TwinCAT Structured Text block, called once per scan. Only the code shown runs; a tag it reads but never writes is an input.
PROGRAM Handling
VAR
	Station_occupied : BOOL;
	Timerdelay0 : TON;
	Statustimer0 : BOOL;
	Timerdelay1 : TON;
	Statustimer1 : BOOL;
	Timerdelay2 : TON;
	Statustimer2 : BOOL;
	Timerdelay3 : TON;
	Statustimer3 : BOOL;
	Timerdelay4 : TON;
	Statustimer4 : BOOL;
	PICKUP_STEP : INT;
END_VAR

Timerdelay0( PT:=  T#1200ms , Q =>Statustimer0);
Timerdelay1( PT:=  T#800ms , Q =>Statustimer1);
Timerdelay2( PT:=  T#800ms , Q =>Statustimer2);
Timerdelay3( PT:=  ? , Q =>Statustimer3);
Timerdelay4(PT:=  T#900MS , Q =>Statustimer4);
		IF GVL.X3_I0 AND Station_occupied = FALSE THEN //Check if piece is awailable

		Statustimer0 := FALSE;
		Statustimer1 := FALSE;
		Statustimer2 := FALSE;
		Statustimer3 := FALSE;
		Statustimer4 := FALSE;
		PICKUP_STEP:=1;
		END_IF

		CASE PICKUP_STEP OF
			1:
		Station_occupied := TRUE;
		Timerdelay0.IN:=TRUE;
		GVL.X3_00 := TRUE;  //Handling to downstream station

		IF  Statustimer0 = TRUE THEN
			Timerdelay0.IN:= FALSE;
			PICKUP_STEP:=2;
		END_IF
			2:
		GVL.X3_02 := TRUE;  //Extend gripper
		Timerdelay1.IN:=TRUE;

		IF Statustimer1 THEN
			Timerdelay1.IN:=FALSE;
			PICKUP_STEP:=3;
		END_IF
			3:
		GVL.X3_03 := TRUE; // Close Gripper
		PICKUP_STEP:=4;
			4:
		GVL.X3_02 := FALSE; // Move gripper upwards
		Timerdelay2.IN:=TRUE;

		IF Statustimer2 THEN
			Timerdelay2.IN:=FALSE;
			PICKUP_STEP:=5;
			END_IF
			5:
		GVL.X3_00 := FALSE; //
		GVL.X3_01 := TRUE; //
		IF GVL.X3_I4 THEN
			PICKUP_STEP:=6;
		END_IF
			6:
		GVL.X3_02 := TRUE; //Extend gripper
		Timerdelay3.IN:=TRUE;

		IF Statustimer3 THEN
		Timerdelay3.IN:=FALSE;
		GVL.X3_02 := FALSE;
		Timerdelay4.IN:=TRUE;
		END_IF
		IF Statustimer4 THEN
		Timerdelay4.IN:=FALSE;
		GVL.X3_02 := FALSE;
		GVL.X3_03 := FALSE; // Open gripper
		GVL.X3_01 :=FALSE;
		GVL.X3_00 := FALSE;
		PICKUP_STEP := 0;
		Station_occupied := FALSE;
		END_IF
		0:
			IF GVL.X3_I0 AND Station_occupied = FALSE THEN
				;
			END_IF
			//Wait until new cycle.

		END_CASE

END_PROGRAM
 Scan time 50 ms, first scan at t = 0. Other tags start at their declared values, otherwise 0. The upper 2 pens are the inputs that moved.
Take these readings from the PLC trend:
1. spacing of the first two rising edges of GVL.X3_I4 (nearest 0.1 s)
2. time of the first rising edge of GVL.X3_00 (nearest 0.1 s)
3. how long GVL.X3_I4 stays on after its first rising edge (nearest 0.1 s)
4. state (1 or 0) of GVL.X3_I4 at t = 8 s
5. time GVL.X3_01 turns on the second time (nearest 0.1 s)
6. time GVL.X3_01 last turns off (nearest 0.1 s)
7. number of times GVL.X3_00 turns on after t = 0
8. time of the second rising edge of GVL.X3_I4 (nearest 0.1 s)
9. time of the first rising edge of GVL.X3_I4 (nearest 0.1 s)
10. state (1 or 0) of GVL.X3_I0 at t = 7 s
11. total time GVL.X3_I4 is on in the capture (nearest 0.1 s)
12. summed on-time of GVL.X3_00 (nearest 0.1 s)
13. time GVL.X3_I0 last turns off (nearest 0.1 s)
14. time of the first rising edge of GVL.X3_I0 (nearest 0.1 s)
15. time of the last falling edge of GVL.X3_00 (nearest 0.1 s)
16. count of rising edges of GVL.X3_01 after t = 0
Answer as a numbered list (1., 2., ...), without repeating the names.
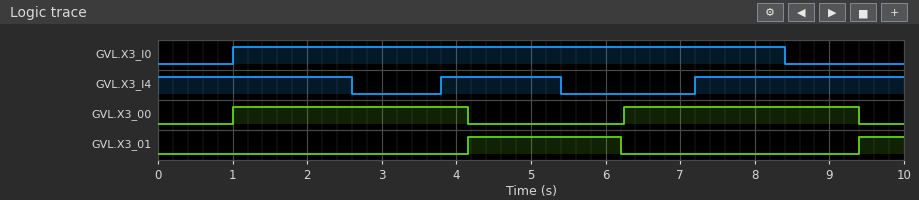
1. 3.4 s
2. 1.0 s
3. 1.6 s
4. 1
5. 9.4 s
6. 6.2 s
7. 2
8. 7.2 s
9. 3.8 s
10. 1
11. 7.0 s
12. 6.3 s
13. 8.4 s
14. 1.0 s
15. 9.4 s
16. 2
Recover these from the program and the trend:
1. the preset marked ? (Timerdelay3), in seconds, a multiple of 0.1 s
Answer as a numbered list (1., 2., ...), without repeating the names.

1. 1.0 s
